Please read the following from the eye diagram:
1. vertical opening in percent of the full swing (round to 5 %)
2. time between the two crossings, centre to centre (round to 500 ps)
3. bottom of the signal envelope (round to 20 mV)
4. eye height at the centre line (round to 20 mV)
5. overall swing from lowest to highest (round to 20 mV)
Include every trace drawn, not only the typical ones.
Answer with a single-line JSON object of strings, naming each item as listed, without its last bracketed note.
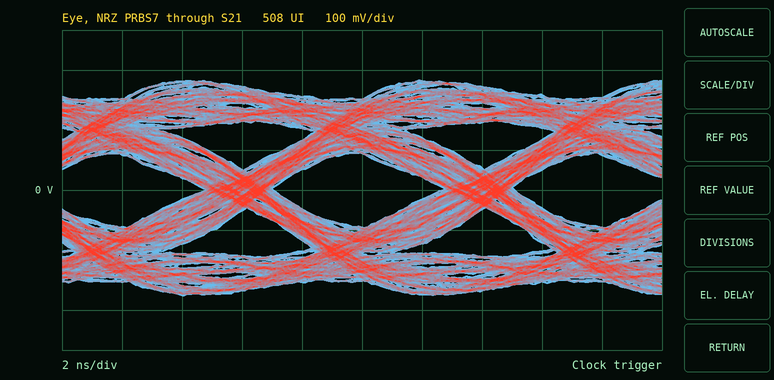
{"vertical opening in percent of the full swing": "35 %", "time between the two crossings, centre to centre": "8.0 ns", "bottom of the signal envelope": "-260 mV", "eye height at the centre line": "180 mV", "overall swing from lowest to highest": "540 mV"}
